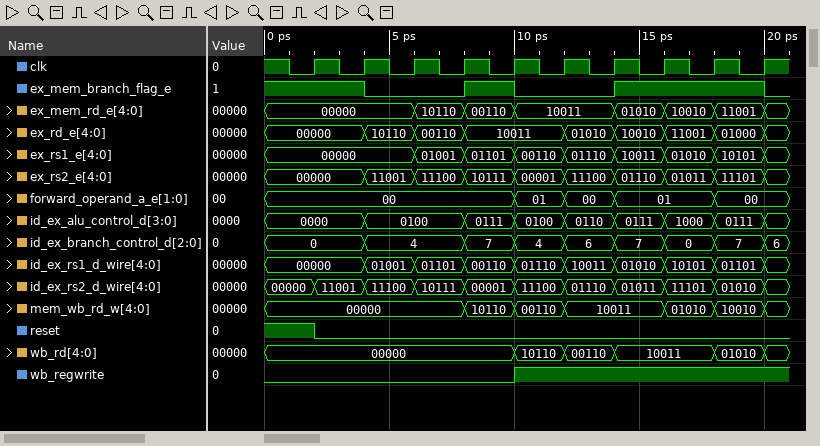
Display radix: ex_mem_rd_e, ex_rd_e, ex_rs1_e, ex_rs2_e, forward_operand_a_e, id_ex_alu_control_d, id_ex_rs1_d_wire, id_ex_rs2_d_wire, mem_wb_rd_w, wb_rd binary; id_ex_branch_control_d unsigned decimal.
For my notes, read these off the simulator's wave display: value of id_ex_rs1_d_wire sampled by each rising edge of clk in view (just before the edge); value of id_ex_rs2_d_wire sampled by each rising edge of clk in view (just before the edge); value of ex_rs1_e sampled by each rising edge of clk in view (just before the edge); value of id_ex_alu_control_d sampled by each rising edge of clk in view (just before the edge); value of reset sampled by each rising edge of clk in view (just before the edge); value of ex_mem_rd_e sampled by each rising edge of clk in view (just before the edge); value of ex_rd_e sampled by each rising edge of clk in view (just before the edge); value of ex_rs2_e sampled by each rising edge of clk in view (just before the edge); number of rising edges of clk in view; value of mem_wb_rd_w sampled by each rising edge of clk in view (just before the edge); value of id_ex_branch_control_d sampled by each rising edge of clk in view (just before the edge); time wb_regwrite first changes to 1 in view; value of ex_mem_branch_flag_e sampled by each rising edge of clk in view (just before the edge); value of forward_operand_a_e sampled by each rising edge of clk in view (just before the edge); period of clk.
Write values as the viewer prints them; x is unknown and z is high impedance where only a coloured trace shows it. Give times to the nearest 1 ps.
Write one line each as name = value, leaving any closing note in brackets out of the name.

value of id_ex_rs1_d_wire sampled by each rising edge of clk in view = 00000, 00000, 01001, 01101, 00110, 01110, 10011, 01010, 10101, 01101
value of id_ex_rs2_d_wire sampled by each rising edge of clk in view = 00000, 11001, 11100, 10111, 00001, 11100, 01110, 01011, 11101, 01010
value of ex_rs1_e sampled by each rising edge of clk in view = 00000, 00000, 00000, 01001, 01101, 00110, 01110, 10011, 01010, 10101
value of id_ex_alu_control_d sampled by each rising edge of clk in view = 0000, 0000, 0100, 0100, 0111, 0100, 0110, 0111, 1000, 0111
value of reset sampled by each rising edge of clk in view = 1 0 0 0 0 0 0 0 0 0
value of ex_mem_rd_e sampled by each rising edge of clk in view = 00000, 00000, 00000, 10110, 00110, 10011, 10011, 01010, 10010, 11001
value of ex_rd_e sampled by each rising edge of clk in view = 00000, 00000, 10110, 00110, 10011, 10011, 01010, 10010, 11001, 01000
value of ex_rs2_e sampled by each rising edge of clk in view = 00000, 00000, 11001, 11100, 10111, 00001, 11100, 01110, 01011, 11101
number of rising edges of clk in view = 10
value of mem_wb_rd_w sampled by each rising edge of clk in view = 00000, 00000, 00000, 00000, 10110, 00110, 10011, 10011, 01010, 10010
value of id_ex_branch_control_d sampled by each rising edge of clk in view = 0, 0, 4, 4, 7, 4, 6, 7, 0, 7
time wb_regwrite first changes to 1 in view = 10 ps
value of ex_mem_branch_flag_e sampled by each rising edge of clk in view = 1 1 0 0 1 0 0 1 1 1
value of forward_operand_a_e sampled by each rising edge of clk in view = 00, 00, 00, 00, 00, 01, 00, 01, 01, 00
period of clk = 2 ps
